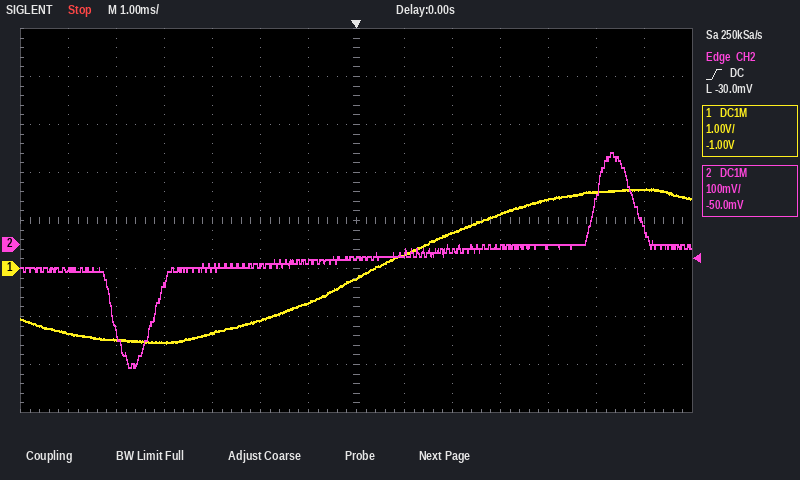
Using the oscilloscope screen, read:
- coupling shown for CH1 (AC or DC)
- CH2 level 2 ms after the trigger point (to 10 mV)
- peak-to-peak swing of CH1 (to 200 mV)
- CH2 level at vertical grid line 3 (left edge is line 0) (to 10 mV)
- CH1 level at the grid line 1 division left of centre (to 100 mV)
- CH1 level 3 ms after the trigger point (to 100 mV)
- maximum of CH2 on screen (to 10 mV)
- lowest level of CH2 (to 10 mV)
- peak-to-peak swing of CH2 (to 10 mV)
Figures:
DC
-10 mV
3.2 V
-80 mV
-700 mV
1.1 V
190 mV
-260 mV
450 mV
